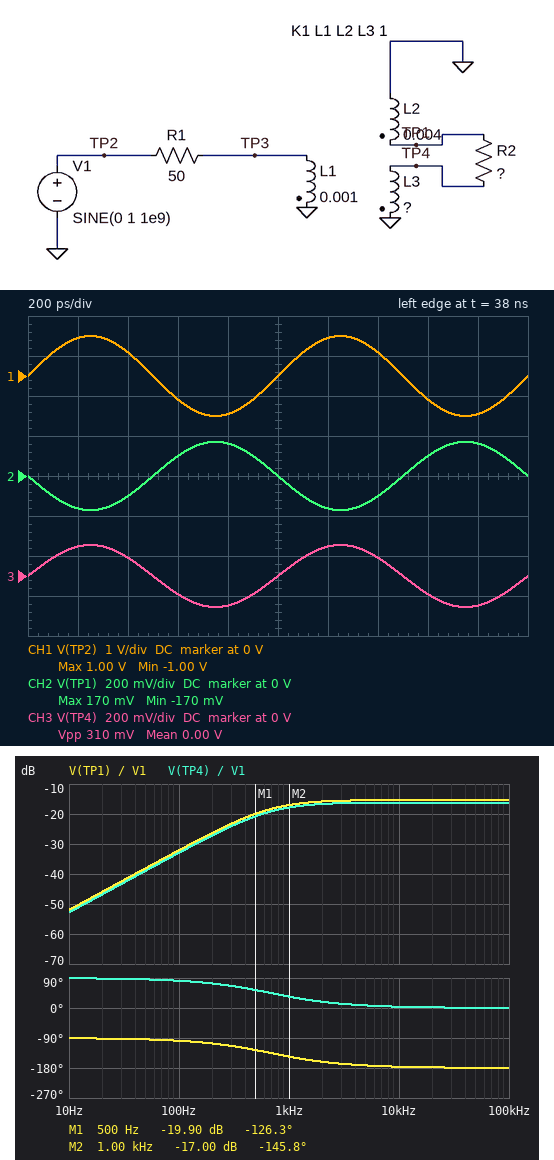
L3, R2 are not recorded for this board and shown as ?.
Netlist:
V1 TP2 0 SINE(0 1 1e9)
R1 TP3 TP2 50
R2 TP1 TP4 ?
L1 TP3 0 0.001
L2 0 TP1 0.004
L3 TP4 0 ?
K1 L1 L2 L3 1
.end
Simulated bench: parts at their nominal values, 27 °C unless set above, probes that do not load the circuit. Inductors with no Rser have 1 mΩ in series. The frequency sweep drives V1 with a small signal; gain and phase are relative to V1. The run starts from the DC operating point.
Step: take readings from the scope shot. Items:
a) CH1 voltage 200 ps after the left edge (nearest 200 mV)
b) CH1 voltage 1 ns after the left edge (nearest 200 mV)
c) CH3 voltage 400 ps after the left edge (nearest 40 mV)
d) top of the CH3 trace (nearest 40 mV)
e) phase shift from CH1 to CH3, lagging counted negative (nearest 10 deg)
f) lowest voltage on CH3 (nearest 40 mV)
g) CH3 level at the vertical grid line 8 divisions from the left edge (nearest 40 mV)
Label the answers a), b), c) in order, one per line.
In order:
a) 1.0 V
b) 0 V
c) 80 mV
d) 160 mV
e) 0 deg
f) -160 mV
g) -80 mV
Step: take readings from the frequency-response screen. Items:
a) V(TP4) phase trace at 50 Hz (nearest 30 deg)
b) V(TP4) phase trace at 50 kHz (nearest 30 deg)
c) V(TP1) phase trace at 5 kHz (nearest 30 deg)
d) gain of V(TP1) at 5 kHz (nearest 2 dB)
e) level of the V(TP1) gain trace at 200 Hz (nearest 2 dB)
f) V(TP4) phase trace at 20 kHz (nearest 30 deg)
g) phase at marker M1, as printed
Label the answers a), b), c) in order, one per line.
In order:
a) 90 deg
b) 0 deg
c) -180 deg
d) -16 dB
e) -26 dB
f) 0 deg
g) -126.3 deg
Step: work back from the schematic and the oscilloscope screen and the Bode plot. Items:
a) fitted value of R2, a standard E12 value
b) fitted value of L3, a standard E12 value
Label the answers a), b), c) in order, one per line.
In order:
a) 68 Ω
b) 3.3 mH
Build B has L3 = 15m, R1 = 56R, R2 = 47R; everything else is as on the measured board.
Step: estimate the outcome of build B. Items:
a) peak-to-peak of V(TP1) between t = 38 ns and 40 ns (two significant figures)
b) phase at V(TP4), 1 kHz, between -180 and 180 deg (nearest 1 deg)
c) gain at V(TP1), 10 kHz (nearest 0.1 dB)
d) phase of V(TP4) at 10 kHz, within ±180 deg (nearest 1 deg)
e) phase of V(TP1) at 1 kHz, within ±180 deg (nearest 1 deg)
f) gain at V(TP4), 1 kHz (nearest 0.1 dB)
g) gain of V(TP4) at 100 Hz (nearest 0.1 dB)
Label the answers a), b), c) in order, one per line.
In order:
a) 95 mV
b) 12 deg
c) -26.5 dB
d) 1 deg
e) -168 deg
f) -20.9 dB
g) -28.1 dB
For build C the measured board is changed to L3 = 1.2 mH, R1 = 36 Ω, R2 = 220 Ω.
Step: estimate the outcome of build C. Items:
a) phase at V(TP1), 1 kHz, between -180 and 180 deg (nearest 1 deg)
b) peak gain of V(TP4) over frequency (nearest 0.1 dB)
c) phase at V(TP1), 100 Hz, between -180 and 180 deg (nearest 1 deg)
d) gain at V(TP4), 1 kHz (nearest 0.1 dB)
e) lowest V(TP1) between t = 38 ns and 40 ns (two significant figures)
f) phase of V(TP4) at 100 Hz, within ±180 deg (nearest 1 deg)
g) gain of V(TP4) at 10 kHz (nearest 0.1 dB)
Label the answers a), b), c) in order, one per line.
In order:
a) -114 deg
b) -7.4 dB
c) -93 deg
d) -15.2 dB
e) -780 mV
f) 87 deg
g) -7.6 dB
